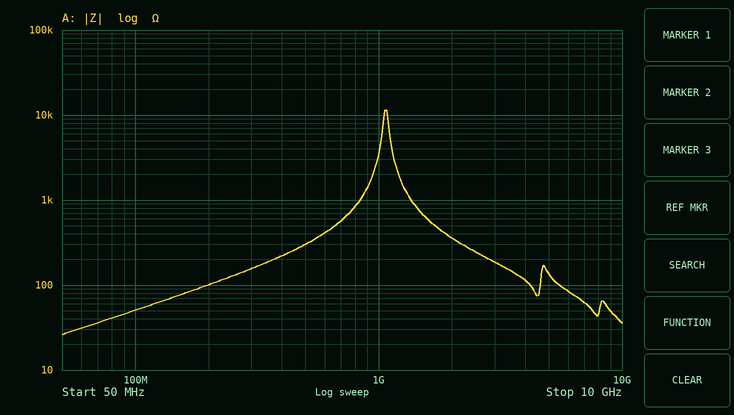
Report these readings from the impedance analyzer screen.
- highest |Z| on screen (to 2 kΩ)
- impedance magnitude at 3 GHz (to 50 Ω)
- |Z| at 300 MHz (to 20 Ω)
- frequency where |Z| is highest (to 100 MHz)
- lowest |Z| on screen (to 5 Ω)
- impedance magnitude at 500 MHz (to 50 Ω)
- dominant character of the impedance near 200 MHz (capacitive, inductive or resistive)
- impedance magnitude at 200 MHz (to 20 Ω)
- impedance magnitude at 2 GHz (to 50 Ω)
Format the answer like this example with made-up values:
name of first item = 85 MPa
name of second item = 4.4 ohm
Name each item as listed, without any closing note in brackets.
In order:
highest |Z| on screen = 12 kΩ
impedance magnitude at 3 GHz = 200 Ω
|Z| at 300 MHz = 160 Ω
frequency where |Z| is highest = 1.1 GHz
lowest |Z| on screen = 25 Ω
impedance magnitude at 500 MHz = 300 Ω
dominant character of the impedance near 200 MHz = inductive
impedance magnitude at 200 MHz = 100 Ω
impedance magnitude at 2 GHz = 350 Ω
